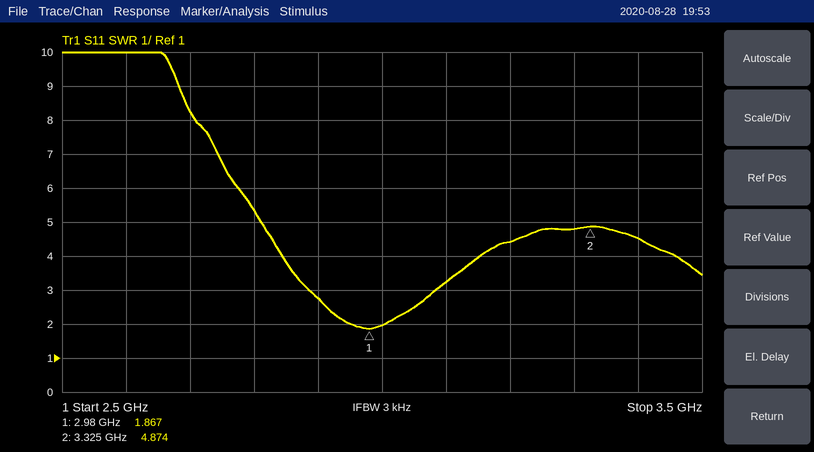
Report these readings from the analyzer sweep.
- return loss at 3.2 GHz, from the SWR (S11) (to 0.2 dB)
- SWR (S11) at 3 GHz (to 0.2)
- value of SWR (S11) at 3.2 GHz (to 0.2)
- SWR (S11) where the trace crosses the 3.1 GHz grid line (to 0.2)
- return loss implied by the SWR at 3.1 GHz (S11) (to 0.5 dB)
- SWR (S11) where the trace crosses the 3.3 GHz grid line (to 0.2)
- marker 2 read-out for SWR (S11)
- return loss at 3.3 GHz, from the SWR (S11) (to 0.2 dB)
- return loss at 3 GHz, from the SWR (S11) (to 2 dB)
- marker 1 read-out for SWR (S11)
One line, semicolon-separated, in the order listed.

4.0 dB; 2.0; 4.4; 3.2; 5.5 dB; 4.8; 4.874; 3.6 dB; 10 dB; 1.867
